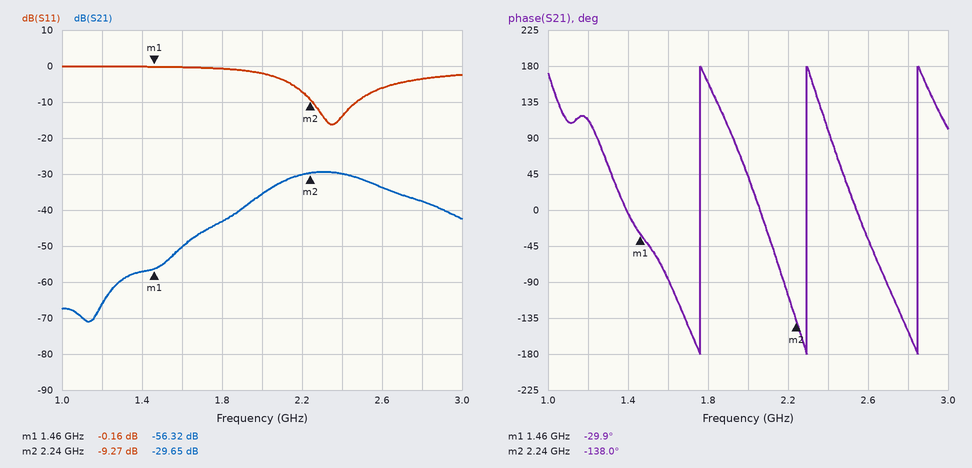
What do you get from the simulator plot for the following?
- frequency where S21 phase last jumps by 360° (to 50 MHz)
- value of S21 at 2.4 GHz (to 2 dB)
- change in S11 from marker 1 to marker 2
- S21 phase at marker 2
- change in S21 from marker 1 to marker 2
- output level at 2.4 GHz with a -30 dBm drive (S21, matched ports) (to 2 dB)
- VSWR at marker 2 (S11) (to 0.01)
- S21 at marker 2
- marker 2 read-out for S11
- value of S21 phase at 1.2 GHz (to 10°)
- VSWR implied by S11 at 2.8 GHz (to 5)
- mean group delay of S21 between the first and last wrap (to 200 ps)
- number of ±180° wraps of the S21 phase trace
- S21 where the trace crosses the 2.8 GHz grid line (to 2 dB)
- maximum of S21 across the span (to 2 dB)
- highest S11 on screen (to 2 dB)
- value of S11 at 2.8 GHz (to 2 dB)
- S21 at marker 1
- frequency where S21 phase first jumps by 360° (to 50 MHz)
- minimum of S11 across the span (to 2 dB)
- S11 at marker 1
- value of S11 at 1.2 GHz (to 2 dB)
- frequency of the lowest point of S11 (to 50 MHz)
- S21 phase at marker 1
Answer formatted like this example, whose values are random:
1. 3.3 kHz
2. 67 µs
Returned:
1. 2.85 GHz
2. -30 dB
3. -9.11 dB
4. -138.0°
5. 26.67 dB
6. -60 dBm
7. 2.05
8. -29.65 dB
9. -9.27 dB
10. 110°
11. 5
12. 1.8 ns
13. 3
14. -38 dB
15. -30 dB
16. 0 dB
17. -4 dB
18. -56.32 dB
19. 1.75 GHz
20. -16 dB
21. -0.16 dB
22. 0 dB
23. 2.35 GHz
24. -29.9°
